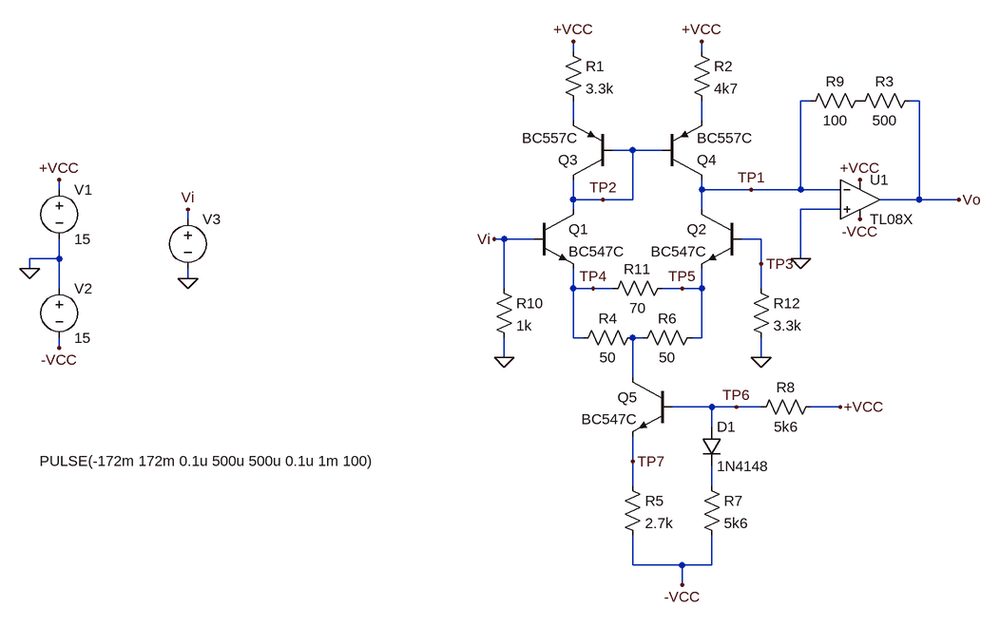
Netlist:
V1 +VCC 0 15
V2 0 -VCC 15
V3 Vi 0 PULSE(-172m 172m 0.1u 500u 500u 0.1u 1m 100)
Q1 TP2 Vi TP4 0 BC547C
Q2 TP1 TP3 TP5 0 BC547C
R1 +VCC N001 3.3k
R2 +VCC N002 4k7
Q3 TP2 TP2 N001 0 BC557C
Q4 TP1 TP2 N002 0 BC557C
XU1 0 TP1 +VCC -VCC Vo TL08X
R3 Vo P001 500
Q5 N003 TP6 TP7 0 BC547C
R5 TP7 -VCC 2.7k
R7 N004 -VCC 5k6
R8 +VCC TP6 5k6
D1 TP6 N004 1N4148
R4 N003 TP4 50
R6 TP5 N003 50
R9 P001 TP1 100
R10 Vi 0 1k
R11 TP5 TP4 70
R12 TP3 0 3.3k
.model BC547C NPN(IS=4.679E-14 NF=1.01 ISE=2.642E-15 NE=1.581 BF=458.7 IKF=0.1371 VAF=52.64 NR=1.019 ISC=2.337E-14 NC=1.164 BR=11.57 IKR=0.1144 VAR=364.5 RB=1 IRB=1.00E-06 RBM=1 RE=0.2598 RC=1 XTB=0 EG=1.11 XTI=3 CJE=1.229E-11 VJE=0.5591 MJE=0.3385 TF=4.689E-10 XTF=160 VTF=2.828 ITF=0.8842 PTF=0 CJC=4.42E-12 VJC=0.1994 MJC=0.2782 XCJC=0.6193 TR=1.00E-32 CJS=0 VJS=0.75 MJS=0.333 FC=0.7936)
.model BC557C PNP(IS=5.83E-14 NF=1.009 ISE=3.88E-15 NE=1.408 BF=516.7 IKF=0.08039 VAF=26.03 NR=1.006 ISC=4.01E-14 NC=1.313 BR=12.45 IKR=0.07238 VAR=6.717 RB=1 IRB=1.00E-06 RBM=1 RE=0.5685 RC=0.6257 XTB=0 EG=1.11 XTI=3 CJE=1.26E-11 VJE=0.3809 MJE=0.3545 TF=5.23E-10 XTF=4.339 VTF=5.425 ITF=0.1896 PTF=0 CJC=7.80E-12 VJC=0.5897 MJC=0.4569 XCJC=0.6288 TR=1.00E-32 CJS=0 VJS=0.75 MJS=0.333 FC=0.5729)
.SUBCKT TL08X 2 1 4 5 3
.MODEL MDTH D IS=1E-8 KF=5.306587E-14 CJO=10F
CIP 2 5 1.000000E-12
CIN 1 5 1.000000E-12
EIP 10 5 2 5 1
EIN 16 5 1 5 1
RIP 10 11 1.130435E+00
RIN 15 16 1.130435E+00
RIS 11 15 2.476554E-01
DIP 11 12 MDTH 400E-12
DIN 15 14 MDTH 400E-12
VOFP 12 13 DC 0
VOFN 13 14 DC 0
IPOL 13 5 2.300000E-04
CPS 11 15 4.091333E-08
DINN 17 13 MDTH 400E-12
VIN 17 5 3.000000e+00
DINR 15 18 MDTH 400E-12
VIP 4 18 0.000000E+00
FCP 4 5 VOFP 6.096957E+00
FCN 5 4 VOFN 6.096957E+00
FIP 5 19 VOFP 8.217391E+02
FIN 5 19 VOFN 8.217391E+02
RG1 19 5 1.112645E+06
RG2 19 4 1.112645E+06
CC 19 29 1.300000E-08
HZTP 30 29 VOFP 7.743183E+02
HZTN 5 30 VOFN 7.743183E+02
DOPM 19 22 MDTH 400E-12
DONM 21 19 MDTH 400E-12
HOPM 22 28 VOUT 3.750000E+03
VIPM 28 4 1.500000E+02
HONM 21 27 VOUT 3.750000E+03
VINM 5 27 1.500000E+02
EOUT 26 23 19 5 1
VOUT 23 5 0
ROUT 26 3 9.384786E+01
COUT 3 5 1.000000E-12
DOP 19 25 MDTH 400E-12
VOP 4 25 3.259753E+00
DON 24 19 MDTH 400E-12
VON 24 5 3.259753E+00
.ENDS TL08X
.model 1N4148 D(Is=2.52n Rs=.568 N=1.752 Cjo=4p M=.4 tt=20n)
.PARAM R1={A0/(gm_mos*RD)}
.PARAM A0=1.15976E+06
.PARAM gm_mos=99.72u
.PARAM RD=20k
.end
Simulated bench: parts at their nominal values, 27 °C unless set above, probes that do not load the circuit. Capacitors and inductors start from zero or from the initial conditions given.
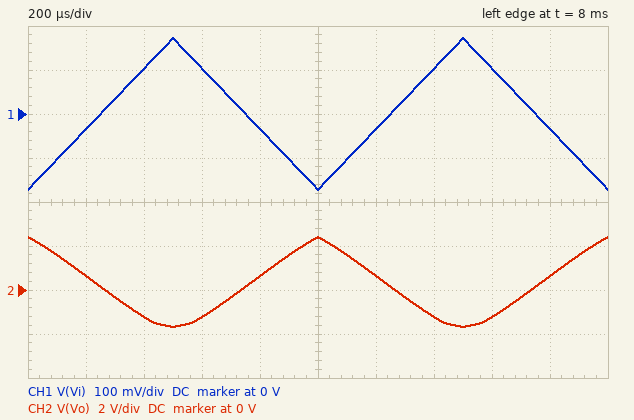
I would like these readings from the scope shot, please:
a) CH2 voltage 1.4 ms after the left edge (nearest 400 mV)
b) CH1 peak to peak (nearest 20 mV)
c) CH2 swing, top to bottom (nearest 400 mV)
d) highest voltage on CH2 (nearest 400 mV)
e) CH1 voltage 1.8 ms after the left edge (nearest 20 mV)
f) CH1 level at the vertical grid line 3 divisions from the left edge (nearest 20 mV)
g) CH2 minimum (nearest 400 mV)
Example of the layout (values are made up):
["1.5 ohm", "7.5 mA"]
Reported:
["-1.2 V", "340 mV", "4.0 V", "2.4 V", "-40 mV", "100 mV", "-1.6 V"]
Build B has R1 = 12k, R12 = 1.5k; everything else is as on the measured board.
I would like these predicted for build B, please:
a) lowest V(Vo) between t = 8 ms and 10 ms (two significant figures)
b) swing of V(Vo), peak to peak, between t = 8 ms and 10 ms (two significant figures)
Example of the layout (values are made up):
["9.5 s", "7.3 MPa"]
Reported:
["-1.4 V", "3.6 V"]
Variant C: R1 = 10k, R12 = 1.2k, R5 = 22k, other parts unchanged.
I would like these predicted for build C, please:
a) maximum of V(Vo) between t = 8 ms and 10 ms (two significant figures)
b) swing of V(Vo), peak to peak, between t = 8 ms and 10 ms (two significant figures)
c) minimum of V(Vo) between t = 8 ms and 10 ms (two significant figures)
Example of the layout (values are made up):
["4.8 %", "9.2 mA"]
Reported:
["320 mV", "1.1 V", "-760 mV"]
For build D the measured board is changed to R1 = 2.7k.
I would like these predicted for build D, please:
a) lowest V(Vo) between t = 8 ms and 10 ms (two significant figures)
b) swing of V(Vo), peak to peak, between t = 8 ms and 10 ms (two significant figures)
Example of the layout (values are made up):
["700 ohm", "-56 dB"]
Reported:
["-1.5 V", "4.0 V"]
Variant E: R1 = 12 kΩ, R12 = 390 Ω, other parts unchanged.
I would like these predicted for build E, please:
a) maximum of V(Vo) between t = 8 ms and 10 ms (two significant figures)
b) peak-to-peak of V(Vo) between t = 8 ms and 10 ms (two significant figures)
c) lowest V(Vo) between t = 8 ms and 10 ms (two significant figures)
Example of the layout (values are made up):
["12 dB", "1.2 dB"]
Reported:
["2.3 V", "3.7 V", "-1.4 V"]
